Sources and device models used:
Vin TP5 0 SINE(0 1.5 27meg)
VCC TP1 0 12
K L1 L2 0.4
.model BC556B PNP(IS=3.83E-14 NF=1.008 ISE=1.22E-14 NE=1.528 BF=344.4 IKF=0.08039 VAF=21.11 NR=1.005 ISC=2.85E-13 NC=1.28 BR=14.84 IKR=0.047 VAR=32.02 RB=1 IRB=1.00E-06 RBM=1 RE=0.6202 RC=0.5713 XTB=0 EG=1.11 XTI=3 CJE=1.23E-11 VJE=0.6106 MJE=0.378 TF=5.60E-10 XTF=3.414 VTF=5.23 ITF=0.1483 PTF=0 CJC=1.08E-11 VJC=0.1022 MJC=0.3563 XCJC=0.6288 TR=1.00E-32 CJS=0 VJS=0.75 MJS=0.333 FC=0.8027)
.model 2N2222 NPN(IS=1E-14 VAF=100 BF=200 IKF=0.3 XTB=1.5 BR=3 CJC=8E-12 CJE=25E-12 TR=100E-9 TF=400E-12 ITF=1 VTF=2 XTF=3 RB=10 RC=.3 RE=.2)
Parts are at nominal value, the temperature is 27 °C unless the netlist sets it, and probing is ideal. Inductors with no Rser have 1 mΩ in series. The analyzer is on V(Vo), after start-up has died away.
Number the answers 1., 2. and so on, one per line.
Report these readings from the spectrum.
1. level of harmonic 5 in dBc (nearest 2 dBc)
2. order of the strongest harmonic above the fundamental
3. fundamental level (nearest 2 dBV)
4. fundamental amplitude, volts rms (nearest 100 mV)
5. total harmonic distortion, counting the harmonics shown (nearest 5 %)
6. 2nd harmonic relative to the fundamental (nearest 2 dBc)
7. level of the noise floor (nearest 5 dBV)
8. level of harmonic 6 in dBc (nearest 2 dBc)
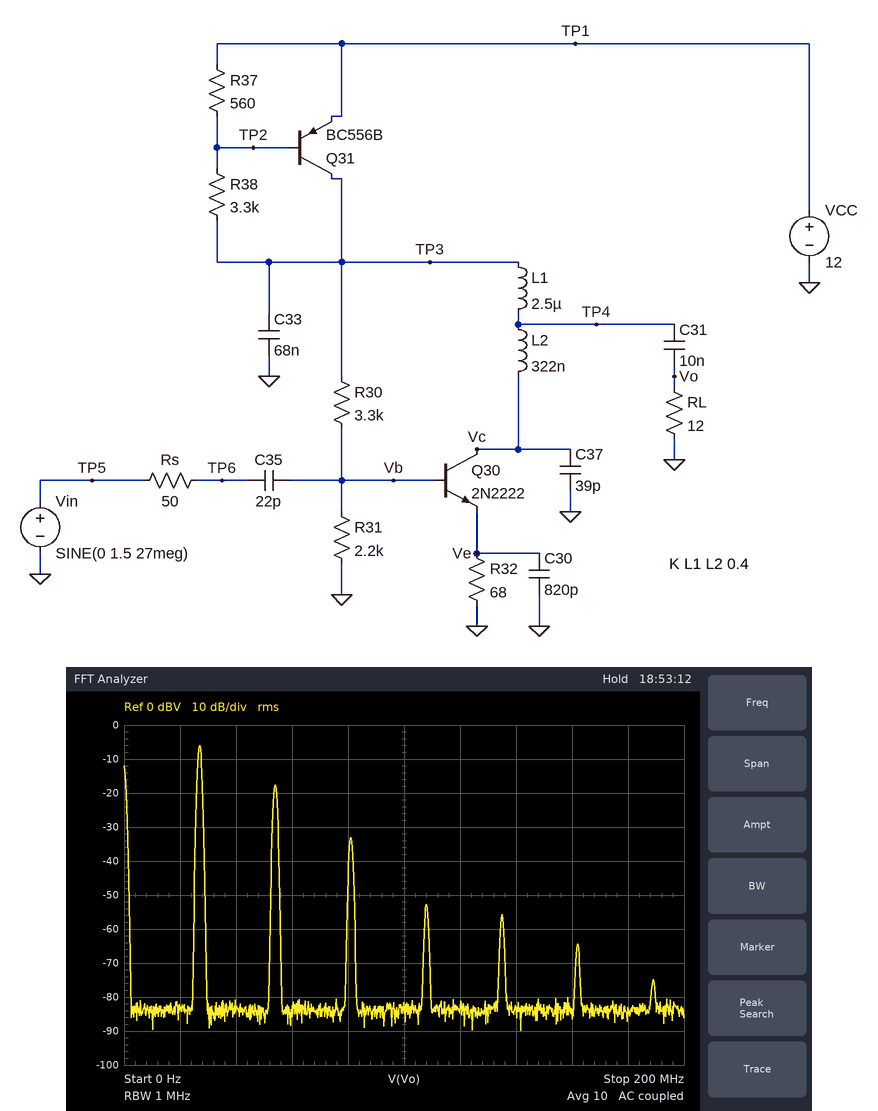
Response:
1. -50 dBc
2. 2
3. -6 dBV
4. 500 mV
5. 25 %
6. -12 dBc
7. -85 dBV
8. -58 dBc
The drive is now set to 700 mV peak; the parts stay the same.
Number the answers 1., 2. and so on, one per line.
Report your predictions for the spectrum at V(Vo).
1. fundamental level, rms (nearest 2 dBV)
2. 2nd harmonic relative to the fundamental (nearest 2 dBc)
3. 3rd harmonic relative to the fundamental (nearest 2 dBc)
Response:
1. -10 dBV
2. -28 dBc
3. -46 dBc
